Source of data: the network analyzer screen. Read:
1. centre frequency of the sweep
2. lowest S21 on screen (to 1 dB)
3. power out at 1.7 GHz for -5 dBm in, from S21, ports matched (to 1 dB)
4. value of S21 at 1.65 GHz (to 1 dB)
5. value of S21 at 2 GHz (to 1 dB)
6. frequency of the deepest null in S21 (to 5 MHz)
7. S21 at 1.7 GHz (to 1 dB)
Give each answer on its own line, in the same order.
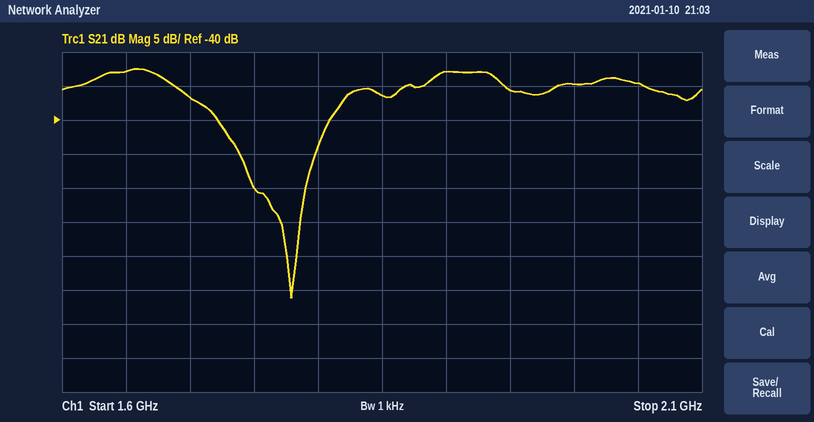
1.85 GHz
-66 dB
-42 dBm
-33 dB
-35 dB
1.780 GHz
-37 dB
